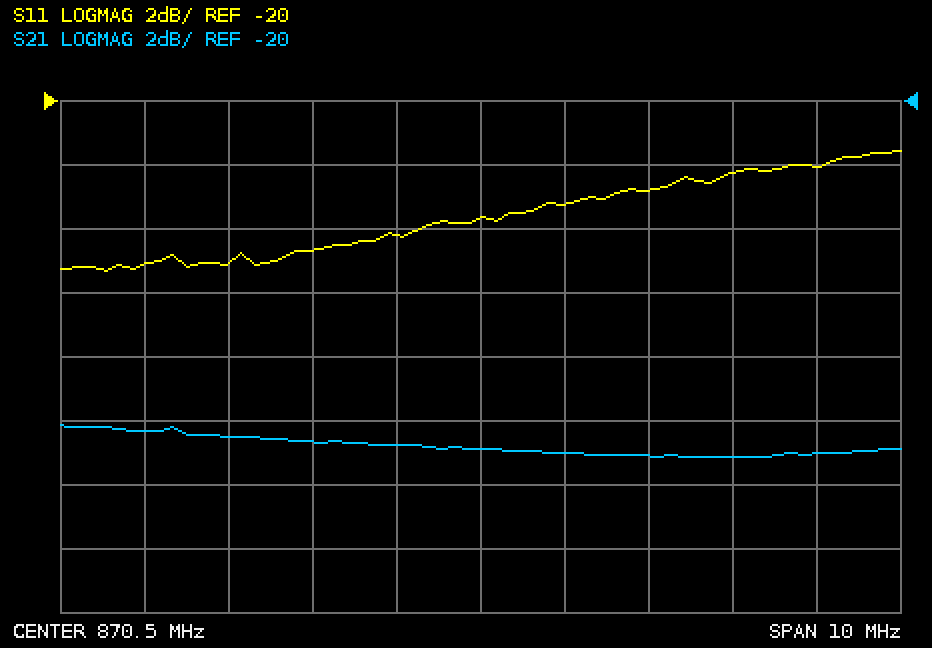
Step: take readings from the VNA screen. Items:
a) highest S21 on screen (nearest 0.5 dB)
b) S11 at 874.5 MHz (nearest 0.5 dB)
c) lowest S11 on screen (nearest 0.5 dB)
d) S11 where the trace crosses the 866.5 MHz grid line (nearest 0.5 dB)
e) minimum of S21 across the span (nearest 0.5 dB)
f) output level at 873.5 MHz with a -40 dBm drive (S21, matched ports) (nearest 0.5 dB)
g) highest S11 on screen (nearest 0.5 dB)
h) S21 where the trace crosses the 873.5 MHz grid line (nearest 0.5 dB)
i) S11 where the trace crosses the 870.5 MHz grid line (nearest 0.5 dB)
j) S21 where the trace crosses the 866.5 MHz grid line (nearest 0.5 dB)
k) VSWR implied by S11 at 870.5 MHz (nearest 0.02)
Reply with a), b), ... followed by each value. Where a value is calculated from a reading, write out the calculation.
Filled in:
a) -30.0 dB
b) -22.0 dB
c) -25.5 dB
d) -25.0 dB
e) -31.0 dB
f) -40 dBm + (-31.0 dB) = -71.0 dBm
g) -21.5 dB
h) -31.0 dB
i) -23.5 dB
j) -30.5 dB
k) |Γ| = 10^(-23.5/20) = 0.0668; VSWR = (1 + 0.0668)/(1 − 0.0668) ≈ 1.14
